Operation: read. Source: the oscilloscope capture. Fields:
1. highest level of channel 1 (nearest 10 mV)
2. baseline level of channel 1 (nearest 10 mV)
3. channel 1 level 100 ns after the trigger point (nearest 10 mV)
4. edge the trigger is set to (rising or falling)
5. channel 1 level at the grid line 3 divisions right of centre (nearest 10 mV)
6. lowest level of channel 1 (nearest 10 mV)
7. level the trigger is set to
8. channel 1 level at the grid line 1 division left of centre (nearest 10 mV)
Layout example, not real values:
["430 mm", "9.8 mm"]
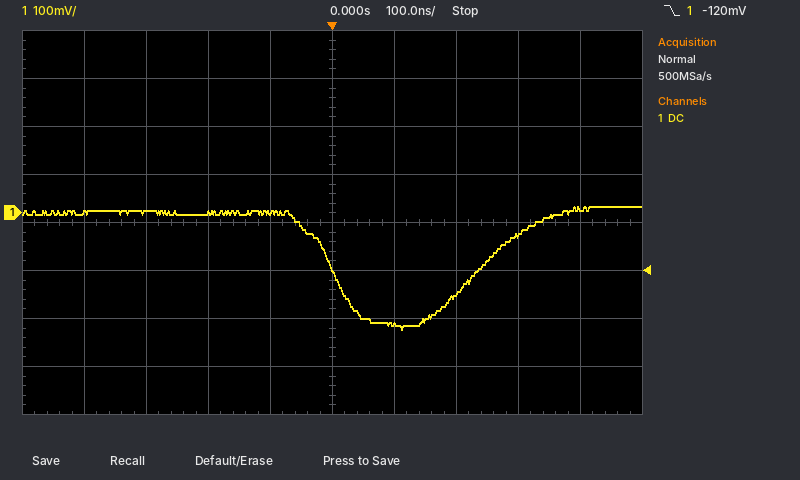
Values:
["10 mV", "0 mV", "-230 mV", "falling", "-50 mV", "-240 mV", "-120 mV", "0 mV"]
